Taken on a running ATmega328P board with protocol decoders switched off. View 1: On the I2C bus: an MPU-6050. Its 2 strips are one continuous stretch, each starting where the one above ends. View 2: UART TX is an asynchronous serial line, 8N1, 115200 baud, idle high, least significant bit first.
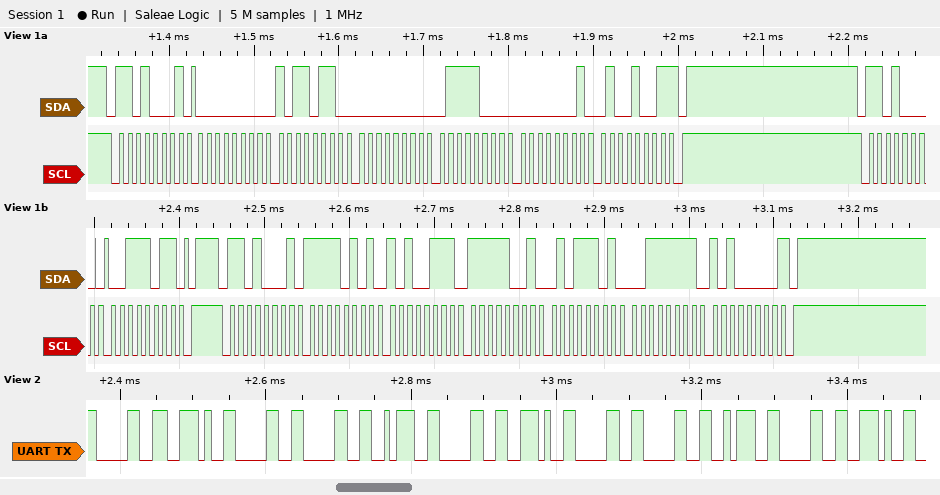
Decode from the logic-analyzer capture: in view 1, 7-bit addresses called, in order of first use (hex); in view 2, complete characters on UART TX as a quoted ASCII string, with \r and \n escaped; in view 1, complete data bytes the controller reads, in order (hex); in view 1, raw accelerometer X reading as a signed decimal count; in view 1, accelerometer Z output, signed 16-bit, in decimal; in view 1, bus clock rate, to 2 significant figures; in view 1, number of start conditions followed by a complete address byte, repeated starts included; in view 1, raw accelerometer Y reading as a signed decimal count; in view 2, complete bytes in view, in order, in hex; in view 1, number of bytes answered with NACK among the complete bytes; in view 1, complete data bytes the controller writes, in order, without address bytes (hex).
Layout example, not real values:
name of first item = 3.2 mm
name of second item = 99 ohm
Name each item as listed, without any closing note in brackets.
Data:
in view 1, 7-bit addresses called, in order of first use = 0x68
in view 2, complete characters on UART TX as a quoted ASCII string, with \r and \n escaped = "0.00:0.00:0."
in view 1, complete data bytes the controller reads, in order = 00 B6 00 78 01 49 F5 A7 F9 5D 3F A0
in view 1, raw accelerometer X reading as a signed decimal count = -2649
in view 1, accelerometer Z output, signed 16-bit, in decimal = 16288
in view 1, bus clock rate, to 2 significant figures = 100 kHz
in view 1, number of start conditions followed by a complete address byte, repeated starts included = 3
in view 1, raw accelerometer Y reading as a signed decimal count = -1699
in view 2, complete bytes in view, in order, in hex = 0x30 0x2E 0x30 0x30 0x3A 0x30 0x2E 0x30 0x30 0x3A 0x30 0x2E
in view 1, number of bytes answered with NACK among the complete bytes = 2
in view 1, complete data bytes the controller writes, in order, without address bytes = 3B
